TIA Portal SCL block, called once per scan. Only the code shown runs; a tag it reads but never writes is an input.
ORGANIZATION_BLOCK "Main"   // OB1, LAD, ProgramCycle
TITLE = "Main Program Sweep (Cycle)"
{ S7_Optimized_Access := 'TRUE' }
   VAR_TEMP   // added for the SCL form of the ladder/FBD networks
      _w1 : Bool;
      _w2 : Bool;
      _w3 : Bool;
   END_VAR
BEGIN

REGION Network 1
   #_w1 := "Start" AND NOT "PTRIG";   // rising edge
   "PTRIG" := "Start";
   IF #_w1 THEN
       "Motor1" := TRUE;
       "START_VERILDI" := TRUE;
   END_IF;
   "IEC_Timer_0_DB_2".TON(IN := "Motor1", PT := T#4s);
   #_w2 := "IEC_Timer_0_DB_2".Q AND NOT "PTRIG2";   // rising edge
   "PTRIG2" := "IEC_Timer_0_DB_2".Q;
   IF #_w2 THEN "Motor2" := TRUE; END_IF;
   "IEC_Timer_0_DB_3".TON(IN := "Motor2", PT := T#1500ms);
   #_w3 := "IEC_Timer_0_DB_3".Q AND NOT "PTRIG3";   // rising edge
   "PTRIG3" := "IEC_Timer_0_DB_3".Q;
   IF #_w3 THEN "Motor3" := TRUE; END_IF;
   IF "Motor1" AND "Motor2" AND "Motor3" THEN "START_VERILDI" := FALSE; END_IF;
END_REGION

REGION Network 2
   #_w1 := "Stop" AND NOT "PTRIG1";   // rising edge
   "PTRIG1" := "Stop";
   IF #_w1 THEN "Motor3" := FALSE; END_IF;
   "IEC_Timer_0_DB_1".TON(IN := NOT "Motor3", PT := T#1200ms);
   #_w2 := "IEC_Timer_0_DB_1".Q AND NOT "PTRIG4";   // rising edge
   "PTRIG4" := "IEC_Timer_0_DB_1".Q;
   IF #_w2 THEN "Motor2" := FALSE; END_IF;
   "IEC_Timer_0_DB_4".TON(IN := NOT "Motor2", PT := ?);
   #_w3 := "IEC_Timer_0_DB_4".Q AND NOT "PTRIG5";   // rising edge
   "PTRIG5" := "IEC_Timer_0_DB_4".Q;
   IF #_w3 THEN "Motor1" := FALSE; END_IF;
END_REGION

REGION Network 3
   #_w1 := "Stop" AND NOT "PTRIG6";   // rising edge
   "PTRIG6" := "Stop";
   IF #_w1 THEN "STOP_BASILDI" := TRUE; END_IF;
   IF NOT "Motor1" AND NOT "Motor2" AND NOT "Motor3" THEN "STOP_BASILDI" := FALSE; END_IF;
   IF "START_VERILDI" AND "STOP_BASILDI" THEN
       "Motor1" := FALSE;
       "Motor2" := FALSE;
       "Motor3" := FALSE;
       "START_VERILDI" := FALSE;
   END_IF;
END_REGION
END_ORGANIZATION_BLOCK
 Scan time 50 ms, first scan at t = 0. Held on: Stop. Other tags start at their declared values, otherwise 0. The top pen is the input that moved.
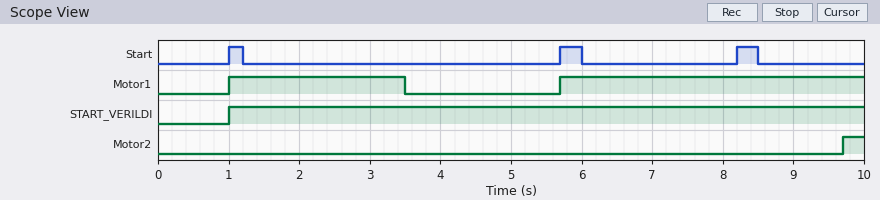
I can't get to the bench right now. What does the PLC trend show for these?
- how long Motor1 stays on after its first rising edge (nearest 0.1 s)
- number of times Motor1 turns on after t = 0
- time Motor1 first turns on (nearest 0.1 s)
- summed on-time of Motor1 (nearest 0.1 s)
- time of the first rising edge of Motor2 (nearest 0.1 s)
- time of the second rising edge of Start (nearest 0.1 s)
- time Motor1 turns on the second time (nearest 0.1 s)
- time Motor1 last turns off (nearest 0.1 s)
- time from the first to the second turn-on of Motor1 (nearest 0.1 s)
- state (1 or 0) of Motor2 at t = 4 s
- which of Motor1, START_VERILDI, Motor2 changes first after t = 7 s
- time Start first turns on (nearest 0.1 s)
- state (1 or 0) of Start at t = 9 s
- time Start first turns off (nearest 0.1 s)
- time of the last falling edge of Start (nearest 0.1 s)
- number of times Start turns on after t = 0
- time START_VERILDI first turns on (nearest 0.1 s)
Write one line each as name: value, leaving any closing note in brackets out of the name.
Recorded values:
how long Motor1 stays on after its first rising edge: 2.5 s
number of times Motor1 turns on after t = 0: 2
time Motor1 first turns on: 1.0 s
summed on-time of Motor1: 6.8 s
time of the first rising edge of Motor2: 9.7 s
time of the second rising edge of Start: 5.7 s
time Motor1 turns on the second time: 5.7 s
time Motor1 last turns off: 3.5 s
time from the first to the second turn-on of Motor1: 4.7 s
state (1 or 0) of Motor2 at t = 4 s: 0
which of Motor1, START_VERILDI, Motor2 changes first after t = 7 s: Motor2
time Start first turns on: 1.0 s
state (1 or 0) of Start at t = 9 s: 0
time Start first turns off: 1.2 s
time of the last falling edge of Start: 8.5 s
number of times Start turns on after t = 0: 3
time START_VERILDI first turns on: 1.0 s
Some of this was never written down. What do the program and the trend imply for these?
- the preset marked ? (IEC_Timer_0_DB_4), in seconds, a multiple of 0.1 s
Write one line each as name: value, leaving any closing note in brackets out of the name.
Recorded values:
the preset marked ? (IEC_Timer_0_DB_4), in seconds, a multiple of 0.1 s: 3.5 s
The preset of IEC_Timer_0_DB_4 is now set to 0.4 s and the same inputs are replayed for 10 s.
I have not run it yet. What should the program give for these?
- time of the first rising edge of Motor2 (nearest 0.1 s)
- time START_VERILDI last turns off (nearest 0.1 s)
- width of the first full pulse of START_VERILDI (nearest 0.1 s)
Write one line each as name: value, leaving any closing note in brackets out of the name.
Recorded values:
time of the first rising edge of Motor2: 5.0 s
time START_VERILDI last turns off: 6.5 s
width of the first full pulse of START_VERILDI: 5.5 s
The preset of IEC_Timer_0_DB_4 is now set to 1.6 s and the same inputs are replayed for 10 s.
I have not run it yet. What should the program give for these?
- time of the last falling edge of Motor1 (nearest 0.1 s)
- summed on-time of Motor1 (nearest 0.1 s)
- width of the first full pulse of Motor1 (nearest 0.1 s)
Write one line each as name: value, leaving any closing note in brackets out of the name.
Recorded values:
time of the last falling edge of Motor1: 1.6 s
summed on-time of Motor1: 4.9 s
width of the first full pulse of Motor1: 0.6 s
